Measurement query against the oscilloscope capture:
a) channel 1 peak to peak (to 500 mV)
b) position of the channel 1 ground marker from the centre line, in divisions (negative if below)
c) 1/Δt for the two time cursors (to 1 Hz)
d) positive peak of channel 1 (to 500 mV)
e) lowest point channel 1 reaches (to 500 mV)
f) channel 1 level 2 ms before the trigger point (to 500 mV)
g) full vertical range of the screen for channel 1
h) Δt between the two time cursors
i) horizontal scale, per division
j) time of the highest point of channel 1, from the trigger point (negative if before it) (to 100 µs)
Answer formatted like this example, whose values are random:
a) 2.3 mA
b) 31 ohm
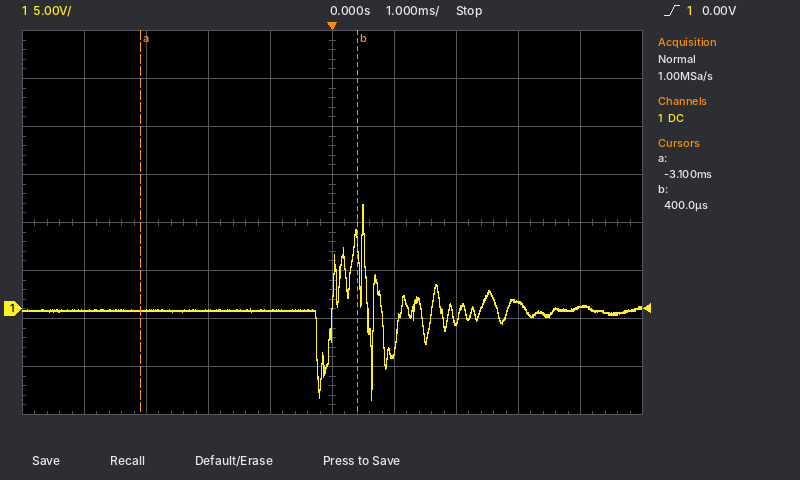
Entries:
a) 20.5 V
b) -1.8 div
c) 286 Hz
d) 11.0 V
e) -9.5 V
f) 0.0 V
g) 40 V
h) 3.5 ms
i) 1 ms
j) +500 µs
